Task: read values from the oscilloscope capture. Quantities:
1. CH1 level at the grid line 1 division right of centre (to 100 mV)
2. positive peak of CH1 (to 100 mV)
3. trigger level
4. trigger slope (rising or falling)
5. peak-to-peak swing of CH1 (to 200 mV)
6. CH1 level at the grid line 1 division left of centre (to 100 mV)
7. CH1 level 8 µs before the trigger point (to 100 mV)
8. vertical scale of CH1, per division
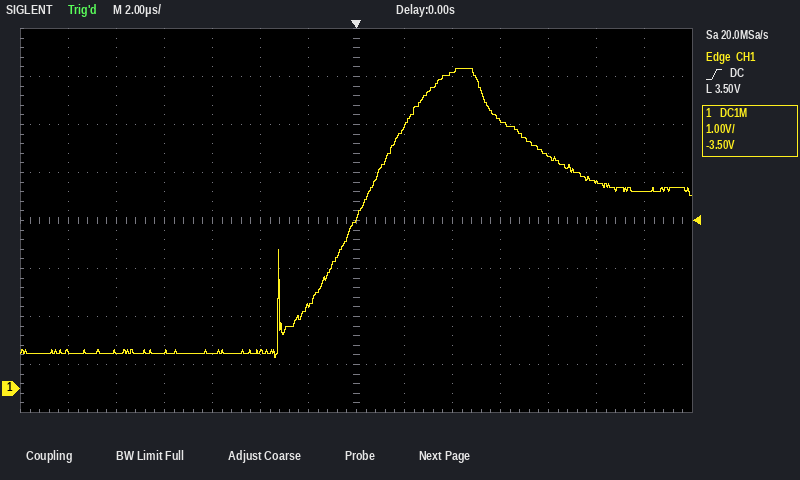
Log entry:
5.5 V
6.7 V
3.50 V
rising
6.0 V
1.7 V
800 mV
1 V
